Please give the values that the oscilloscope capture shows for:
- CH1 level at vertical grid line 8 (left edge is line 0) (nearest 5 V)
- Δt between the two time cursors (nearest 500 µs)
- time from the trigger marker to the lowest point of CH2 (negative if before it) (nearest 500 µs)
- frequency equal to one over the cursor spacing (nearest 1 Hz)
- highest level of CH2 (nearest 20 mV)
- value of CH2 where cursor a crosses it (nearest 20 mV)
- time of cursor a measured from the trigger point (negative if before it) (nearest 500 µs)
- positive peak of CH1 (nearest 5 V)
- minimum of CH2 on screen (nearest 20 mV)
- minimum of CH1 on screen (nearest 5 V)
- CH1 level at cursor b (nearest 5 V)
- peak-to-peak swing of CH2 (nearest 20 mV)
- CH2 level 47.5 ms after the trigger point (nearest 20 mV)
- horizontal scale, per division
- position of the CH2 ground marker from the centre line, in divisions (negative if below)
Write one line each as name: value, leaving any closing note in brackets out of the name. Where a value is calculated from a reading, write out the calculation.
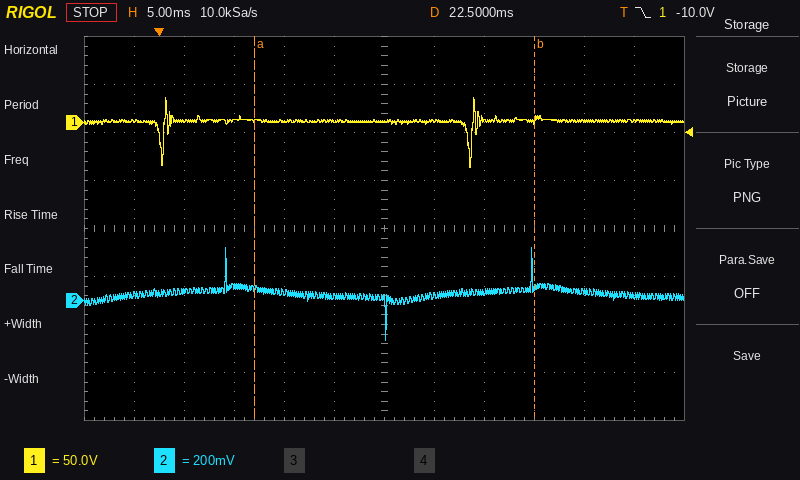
CH1 level at vertical grid line 8 (left edge is line 0): 5 V
Δt between the two time cursors: 28.0 ms
time from the trigger marker to the lowest point of CH2 (negative if before it): +22.5 ms
frequency equal to one over the cursor spacing: 1 / 28.0 ms ≈ 36 Hz
highest level of CH2: 220 mV
value of CH2 where cursor a crosses it: 40 mV
time of cursor a measured from the trigger point (negative if before it): +9.5 ms
positive peak of CH1: 25 V
minimum of CH2 on screen: -160 mV
minimum of CH1 on screen: -45 V
CH1 level at cursor b: 5 V
peak-to-peak swing of CH2: 220 mV − (-160 mV) = 380 mV
CH2 level 47.5 ms after the trigger point: 20 mV
horizontal scale, per division: 5 ms
position of the CH2 ground marker from the centre line, in divisions: -1.5 div
